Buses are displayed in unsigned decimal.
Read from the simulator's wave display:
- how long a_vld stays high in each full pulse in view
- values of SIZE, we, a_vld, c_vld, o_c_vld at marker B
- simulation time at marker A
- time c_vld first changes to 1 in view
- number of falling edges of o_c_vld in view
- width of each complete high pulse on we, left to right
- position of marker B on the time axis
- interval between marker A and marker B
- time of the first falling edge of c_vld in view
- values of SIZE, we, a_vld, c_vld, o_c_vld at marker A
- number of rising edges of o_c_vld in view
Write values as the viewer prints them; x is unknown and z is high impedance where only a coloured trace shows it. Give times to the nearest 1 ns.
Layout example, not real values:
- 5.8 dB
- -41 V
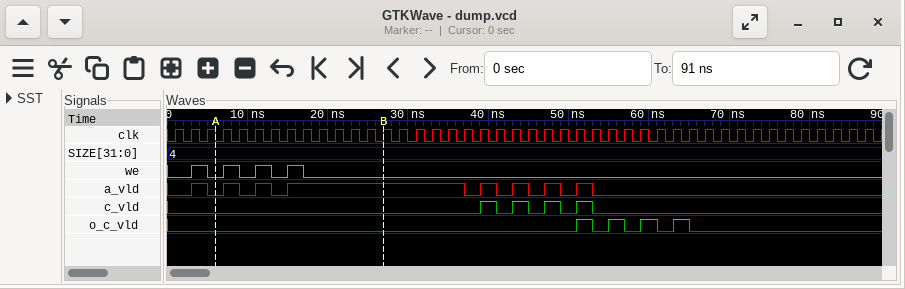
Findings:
- 2 ns, 2 ns, 2 ns, 22 ns, 2 ns, 2 ns, 2 ns, 2 ns
- SIZE=4, we=0, a_vld=1, c_vld=0, o_c_vld=0
- 6 ns
- 39 ns
- 4
- 2 ns, 2 ns, 2 ns, 2 ns
- 27 ns
- 21 ns
- 41 ns
- SIZE=4, we=0, a_vld=0, c_vld=0, o_c_vld=0
- 4
